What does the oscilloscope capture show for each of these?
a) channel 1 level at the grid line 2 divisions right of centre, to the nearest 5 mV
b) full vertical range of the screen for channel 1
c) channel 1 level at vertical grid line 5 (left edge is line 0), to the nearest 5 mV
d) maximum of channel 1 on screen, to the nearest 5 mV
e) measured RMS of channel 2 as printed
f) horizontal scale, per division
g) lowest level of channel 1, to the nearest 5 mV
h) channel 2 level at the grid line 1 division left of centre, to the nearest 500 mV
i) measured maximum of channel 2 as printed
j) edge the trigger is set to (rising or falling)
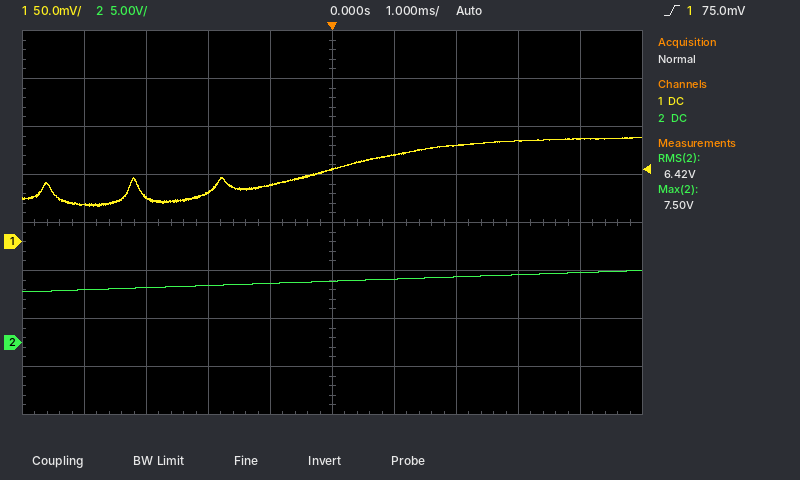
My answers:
100 mV
400 mV
75 mV
110 mV
6.42 V
1 ms
35 mV
6.0 V
7.50 V
rising
